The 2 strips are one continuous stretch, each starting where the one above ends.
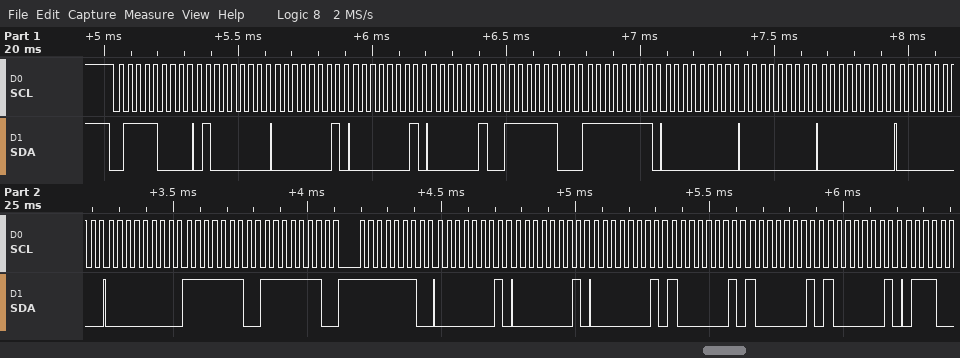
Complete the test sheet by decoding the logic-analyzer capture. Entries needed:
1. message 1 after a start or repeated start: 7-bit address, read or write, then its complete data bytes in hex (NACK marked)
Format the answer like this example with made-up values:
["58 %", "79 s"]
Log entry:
["0x3C write: 40 01 01 02 FC FF 00 00 00 00 00 FE FE FE 01 01 01 81 81 81"]
